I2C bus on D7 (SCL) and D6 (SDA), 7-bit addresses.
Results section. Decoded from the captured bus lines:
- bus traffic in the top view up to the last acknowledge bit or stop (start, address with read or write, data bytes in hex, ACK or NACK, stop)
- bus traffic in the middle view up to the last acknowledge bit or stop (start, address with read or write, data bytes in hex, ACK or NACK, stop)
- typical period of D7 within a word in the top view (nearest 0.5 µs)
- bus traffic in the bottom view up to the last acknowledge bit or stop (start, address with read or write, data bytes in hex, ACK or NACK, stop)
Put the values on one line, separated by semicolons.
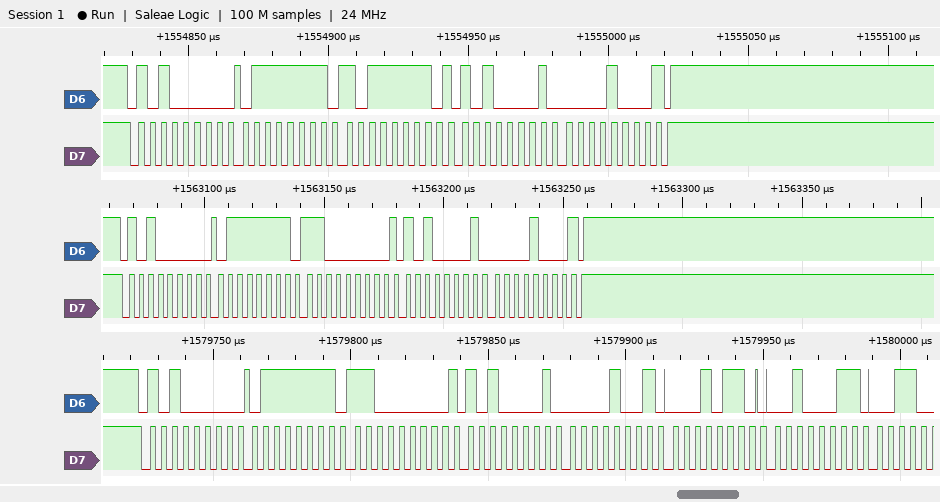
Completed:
start, address 50 write ACK, 7F ACK, BF ACK, repeated start, address 50 read ACK, 08 NACK, stop; start, address 50 write ACK, 7F ACK, C0 ACK, repeated start, address 50 read ACK, 08 NACK, stop; 4 µs; start, address 50 write ACK, 7F ACK, C0 ACK, repeated start, address 50 read ACK, 09 ACK, 16 ACK, 23 ACK
